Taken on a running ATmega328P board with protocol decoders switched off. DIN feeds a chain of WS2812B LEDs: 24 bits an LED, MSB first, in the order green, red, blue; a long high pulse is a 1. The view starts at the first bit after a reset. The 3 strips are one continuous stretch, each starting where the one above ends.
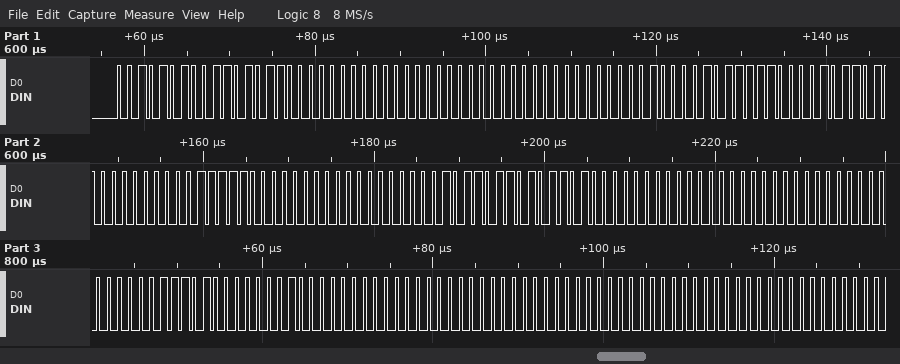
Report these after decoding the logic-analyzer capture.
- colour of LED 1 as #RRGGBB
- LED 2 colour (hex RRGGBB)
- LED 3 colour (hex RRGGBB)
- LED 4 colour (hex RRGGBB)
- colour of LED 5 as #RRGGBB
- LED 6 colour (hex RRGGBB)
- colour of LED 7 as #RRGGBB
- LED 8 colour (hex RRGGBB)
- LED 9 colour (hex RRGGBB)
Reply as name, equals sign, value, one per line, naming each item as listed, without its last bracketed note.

colour of LED 1 as #RRGGBB = #6B2A00
LED 2 colour = #000000
LED 3 colour = #7C212D
LED 4 colour = #3E0000
colour of LED 5 as #RRGGBB = #5B005A
LED 6 colour = #000000
colour of LED 7 as #RRGGBB = #740004
LED 8 colour = #000000
LED 9 colour = #000000
